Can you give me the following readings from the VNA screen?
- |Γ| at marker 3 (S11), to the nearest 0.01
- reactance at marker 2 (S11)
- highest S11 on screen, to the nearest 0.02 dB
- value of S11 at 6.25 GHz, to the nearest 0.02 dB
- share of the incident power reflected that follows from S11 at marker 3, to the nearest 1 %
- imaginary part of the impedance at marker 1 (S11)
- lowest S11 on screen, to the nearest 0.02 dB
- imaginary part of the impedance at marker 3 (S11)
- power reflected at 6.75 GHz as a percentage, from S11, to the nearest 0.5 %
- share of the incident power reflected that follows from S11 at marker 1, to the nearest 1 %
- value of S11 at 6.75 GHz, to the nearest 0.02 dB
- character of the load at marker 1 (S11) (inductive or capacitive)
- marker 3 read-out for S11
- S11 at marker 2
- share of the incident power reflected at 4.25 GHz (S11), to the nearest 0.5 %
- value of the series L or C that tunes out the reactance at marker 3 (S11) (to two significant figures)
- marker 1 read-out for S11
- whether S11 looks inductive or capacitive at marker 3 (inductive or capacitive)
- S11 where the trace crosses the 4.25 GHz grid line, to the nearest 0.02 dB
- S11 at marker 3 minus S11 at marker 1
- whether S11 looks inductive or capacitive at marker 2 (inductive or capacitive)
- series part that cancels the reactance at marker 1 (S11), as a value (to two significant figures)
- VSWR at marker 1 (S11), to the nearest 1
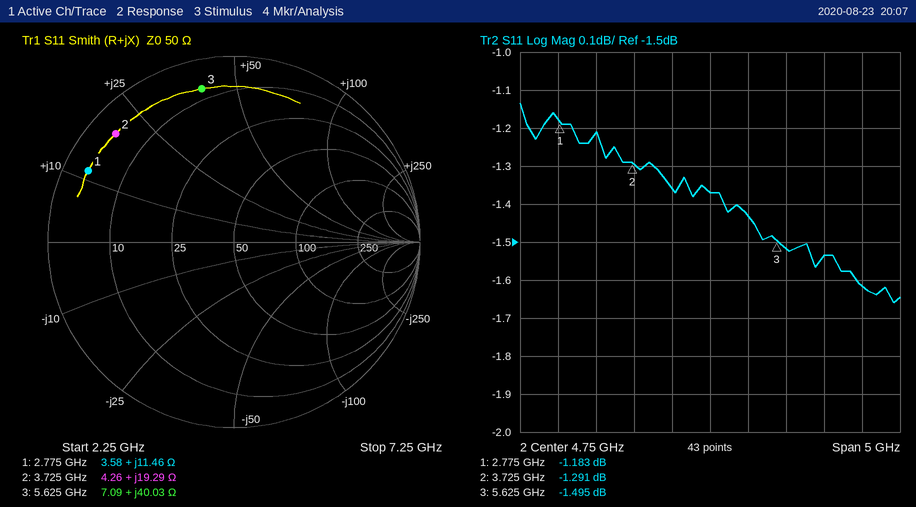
0.84
+19.29 Ω
-1.14 dB
-1.54 dB
71 %
+11.46 Ω
-1.66 dB
+40.03 Ω
69.0 %
76 %
-1.62 dB
inductive
-1.495 dB
-1.291 dB
73.0 %
710 fF
-1.183 dB
inductive
-1.36 dB
-0.312 dB
inductive
5.0 pF
15
